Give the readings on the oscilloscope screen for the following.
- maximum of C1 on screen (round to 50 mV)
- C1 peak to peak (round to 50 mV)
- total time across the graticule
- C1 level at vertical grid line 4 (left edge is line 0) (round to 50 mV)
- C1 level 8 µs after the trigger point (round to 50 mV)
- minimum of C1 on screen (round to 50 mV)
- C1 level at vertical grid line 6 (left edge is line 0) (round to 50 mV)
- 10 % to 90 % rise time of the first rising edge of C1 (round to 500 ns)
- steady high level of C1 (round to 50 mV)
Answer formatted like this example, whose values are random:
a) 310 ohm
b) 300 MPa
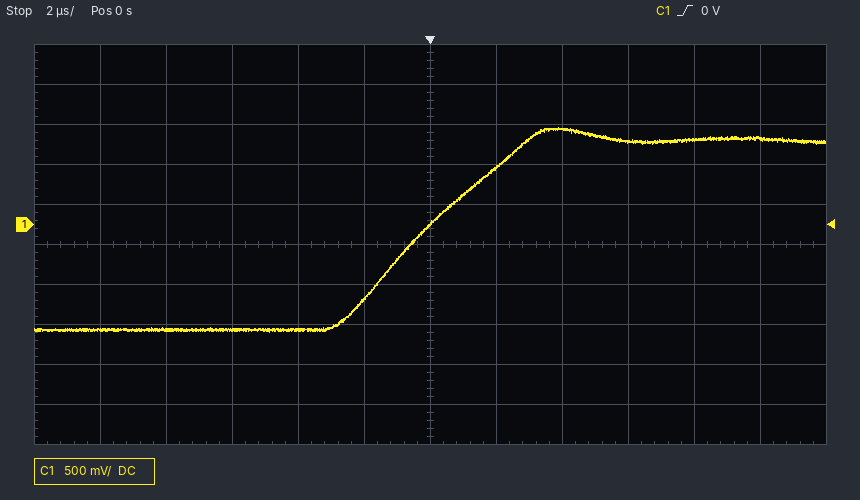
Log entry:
a) 1.20 V
b) 2.55 V
c) 24 µs
d) -1.30 V
e) 1.05 V
f) -1.35 V
g) 0 mV
h) 4.5 µs
i) 1.05 V
